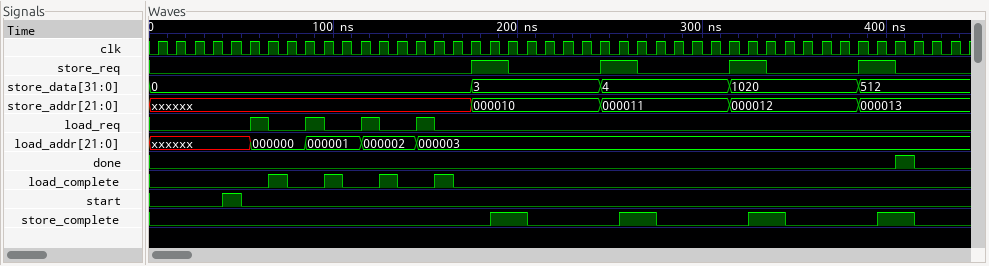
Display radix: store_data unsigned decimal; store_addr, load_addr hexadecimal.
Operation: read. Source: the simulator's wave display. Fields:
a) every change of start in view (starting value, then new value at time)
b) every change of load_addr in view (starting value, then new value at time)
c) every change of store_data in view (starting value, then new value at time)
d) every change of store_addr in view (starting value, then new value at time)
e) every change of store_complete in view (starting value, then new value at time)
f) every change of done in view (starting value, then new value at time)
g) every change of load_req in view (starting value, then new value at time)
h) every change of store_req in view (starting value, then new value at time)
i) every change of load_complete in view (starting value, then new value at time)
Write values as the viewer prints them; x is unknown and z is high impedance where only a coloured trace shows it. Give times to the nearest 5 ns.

0, 1 at 40 ns, 0 at 50 ns
xxxxxx, 000000 at 55 ns, 000001 at 85 ns, 000002 at 115 ns, 000003 at 145 ns
0, 3 at 175 ns, 4 at 245 ns, 1020 at 315 ns, 512 at 385 ns
xxxxxx, 000010 at 175 ns, 000011 at 245 ns, 000012 at 315 ns, 000013 at 385 ns
0, 1 at 185 ns, 0 at 205 ns, 1 at 255 ns, 0 at 275 ns, 1 at 325 ns, 0 at 345 ns, 1 at 395 ns, 0 at 415 ns
0, 1 at 405 ns, 0 at 415 ns
0, 1 at 55 ns, 0 at 65 ns, 1 at 85 ns, 0 at 95 ns, 1 at 115 ns, 0 at 125 ns, 1 at 145 ns, 0 at 155 ns
0, 1 at 175 ns, 0 at 195 ns, 1 at 245 ns, 0 at 265 ns, 1 at 315 ns, 0 at 335 ns, 1 at 385 ns, 0 at 405 ns
0, 1 at 65 ns, 0 at 75 ns, 1 at 95 ns, 0 at 105 ns, 1 at 125 ns, 0 at 135 ns, 1 at 155 ns, 0 at 165 ns
